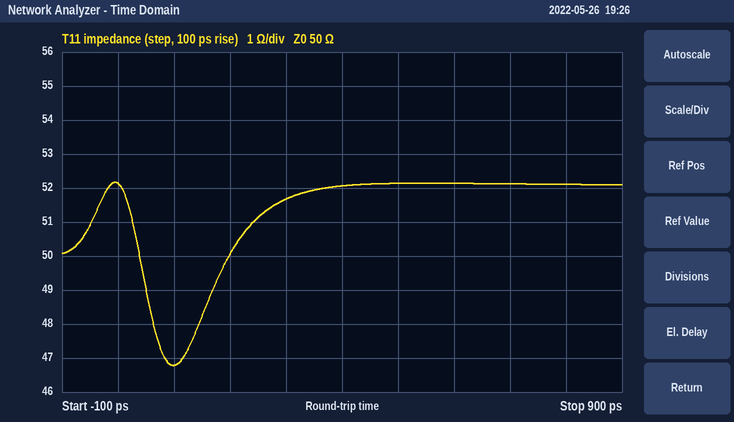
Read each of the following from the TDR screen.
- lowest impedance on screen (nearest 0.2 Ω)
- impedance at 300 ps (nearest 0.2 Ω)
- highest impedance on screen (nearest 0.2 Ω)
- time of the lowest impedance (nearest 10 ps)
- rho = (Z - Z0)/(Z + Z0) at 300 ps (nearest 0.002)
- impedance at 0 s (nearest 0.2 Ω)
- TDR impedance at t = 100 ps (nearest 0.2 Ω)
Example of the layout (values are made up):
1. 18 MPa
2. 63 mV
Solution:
1. 46.8 Ω
2. 51.6 Ω
3. 52.2 Ω
4. 100 ps
5. +0.016
6. 52.2 Ω
7. 46.8 Ω
